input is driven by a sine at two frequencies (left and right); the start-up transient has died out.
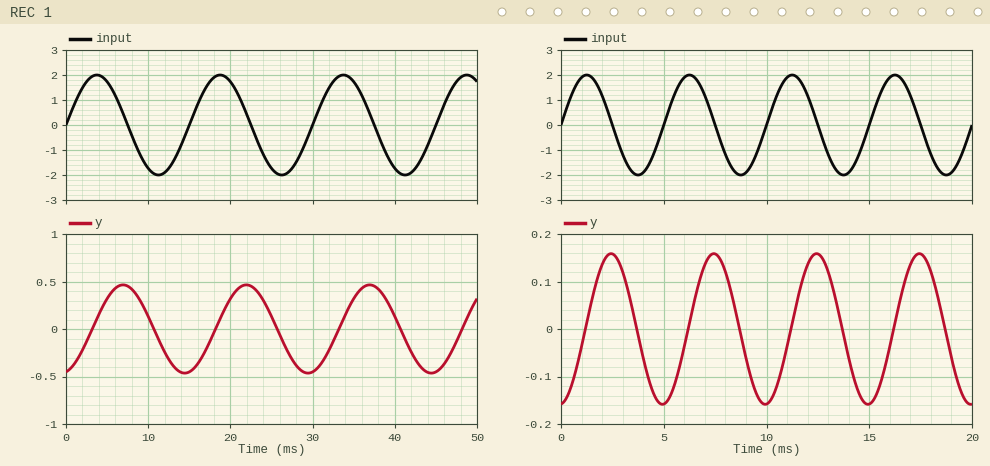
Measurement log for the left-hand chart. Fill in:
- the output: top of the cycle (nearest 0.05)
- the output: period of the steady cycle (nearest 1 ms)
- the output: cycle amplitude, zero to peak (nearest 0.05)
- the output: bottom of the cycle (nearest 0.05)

0.45
15 ms
0.45
-0.45
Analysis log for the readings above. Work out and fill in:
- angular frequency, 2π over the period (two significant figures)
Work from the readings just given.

0.42 rad/ms
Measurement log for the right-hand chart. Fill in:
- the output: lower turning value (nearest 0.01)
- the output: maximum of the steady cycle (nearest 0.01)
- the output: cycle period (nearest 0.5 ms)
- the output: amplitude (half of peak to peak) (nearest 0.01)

-0.16
0.16
5.0 ms
0.16
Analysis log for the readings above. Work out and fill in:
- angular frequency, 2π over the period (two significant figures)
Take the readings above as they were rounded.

1.3 rad/ms
